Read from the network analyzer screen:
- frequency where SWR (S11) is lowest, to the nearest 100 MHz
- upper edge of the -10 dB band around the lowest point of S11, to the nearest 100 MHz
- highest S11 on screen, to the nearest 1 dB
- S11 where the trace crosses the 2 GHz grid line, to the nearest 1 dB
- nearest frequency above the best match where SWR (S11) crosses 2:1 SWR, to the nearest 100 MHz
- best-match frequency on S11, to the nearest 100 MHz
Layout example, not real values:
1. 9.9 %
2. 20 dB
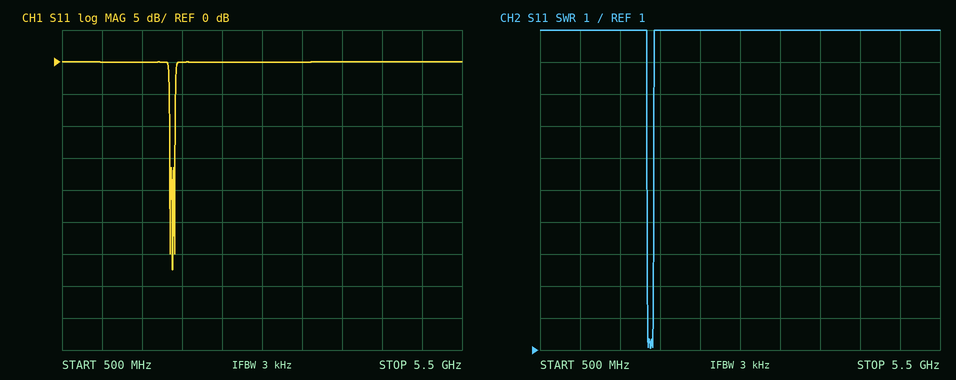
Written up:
1. 1.9 GHz
2. 1.9 GHz
3. 0 dB
4. 0 dB
5. 1.9 GHz
6. 1.9 GHz
